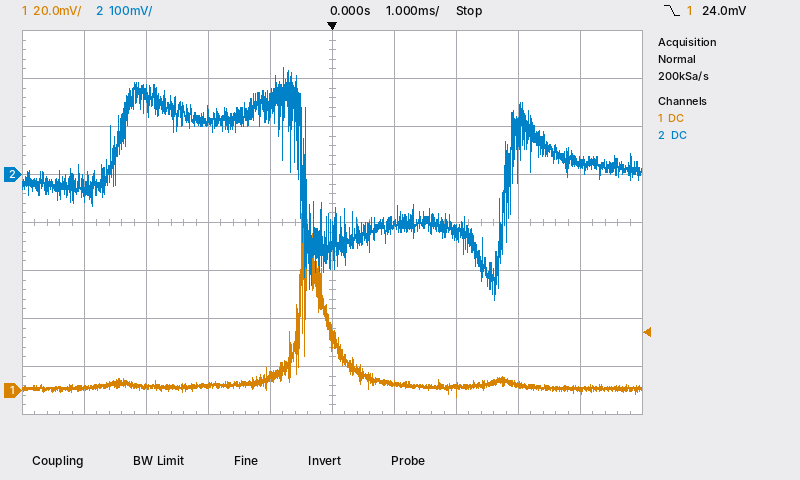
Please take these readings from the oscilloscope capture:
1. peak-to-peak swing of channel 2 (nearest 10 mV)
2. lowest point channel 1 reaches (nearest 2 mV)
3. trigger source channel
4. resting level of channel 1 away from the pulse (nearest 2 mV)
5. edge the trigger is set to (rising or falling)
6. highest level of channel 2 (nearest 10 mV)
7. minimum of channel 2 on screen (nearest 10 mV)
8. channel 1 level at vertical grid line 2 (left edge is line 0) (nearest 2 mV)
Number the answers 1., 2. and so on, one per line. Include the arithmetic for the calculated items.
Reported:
1. 220 mV − (-260 mV) = 480 mV
2. -2 mV
3. channel 1
4. 2 mV
5. falling
6. 220 mV
7. -260 mV
8. 2 mV
